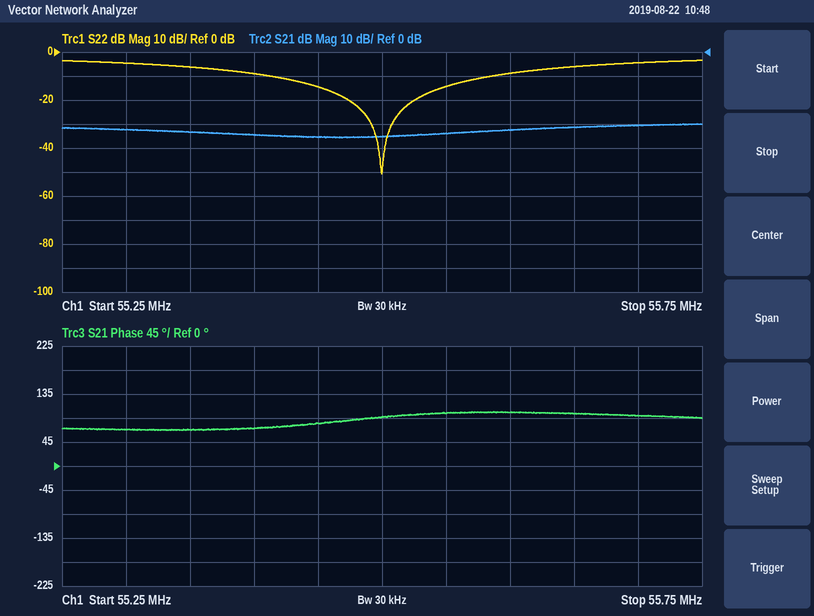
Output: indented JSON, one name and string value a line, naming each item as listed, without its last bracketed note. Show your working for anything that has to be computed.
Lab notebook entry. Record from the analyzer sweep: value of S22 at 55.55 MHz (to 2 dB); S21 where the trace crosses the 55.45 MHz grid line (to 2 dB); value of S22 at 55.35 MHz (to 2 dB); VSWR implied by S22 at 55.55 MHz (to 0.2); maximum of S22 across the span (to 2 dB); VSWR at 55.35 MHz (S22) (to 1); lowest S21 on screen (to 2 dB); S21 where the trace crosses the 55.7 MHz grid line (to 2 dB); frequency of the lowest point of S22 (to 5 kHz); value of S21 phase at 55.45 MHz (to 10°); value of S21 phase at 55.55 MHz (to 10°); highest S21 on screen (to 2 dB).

{
  "value of S22 at 55.55 MHz": "-14 dB",
  "S21 where the trace crosses the 55.45 MHz grid line": "-36 dB",
  "value of S22 at 55.35 MHz": "-6 dB",
  "VSWR implied by S22 at 55.55 MHz": "|Γ| = 10^(-14/20) = 0.1995; VSWR = (1 + 0.1995)/(1 − 0.1995) ≈ 1.50, so 1.4 to the nearest 0.2",
  "maximum of S22 across the span": "-4 dB",
  "VSWR at 55.35 MHz (S22)": "|Γ| = 10^(-6/20) = 0.5012; VSWR = (1 + 0.5012)/(1 − 0.5012) ≈ 3",
  "lowest S21 on screen": "-36 dB",
  "S21 where the trace crosses the 55.7 MHz grid line": "-30 dB",
  "frequency of the lowest point of S22": "55.500 MHz",
  "value of S21 phase at 55.45 MHz": "80°",
  "value of S21 phase at 55.55 MHz": "100°",
  "highest S21 on screen": "-30 dB"
}
